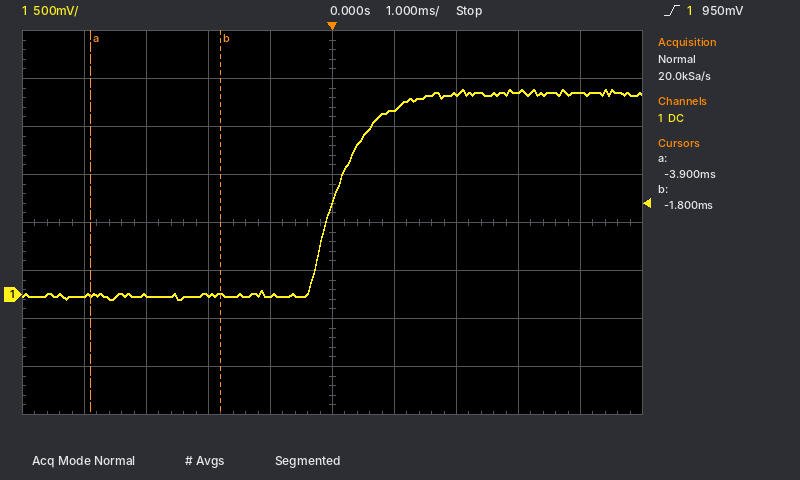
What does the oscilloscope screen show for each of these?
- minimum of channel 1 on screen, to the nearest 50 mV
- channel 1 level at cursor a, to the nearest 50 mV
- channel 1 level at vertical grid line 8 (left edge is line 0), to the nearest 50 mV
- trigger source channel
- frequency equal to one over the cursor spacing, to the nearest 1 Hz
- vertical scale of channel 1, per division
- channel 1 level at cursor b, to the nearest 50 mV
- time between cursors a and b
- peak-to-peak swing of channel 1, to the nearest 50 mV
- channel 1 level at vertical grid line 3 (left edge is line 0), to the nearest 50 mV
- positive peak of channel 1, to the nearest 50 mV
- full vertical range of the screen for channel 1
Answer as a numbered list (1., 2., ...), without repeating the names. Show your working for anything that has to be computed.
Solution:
1. -50 mV
2. 0 mV
3. 2.10 V
4. channel 1
5. 1 / 2.1 ms ≈ 476 Hz
6. 500 mV
7. 0 mV
8. -1.8 ms − (-3.9 ms) = 2.1 ms
9. 2.15 V − (-50 mV) = 2.20 V
10. 0 mV
11. 2.15 V
12. 4 V
